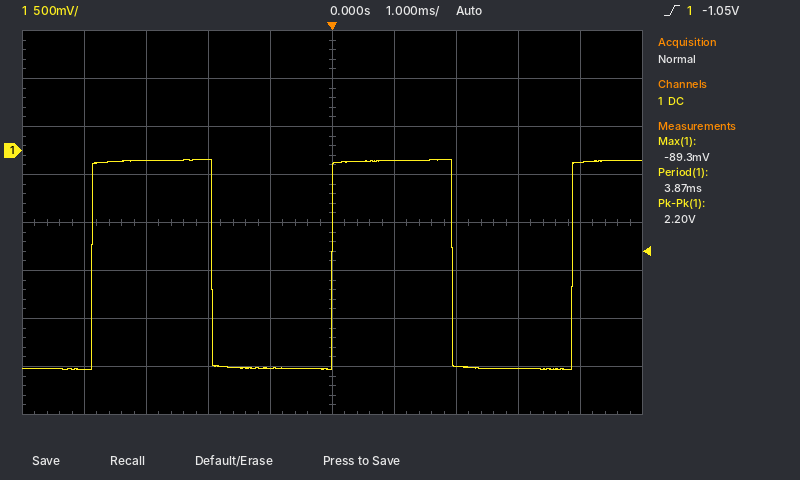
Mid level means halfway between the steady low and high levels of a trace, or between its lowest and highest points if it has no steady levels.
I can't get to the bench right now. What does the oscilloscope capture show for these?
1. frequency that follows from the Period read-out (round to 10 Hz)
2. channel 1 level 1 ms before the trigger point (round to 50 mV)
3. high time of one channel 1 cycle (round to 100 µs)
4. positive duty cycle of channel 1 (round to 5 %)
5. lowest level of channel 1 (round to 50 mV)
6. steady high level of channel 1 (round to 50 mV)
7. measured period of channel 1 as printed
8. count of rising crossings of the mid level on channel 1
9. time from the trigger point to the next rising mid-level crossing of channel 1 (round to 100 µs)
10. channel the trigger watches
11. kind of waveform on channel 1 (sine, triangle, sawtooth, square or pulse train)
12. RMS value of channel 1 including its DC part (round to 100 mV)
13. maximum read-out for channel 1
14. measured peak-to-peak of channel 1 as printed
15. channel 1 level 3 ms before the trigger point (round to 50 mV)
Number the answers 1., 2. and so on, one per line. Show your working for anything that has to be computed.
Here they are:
1. 1 / 3.87 ms ≈ 258 Hz, so 260 Hz to the nearest 10 Hz
2. -2.25 V
3. 1.9 ms
4. 50 %
5. -2.30 V
6. -100 mV
7. 3.87 ms
8. 3
9. 3.9 ms
10. channel 1
11. square
12. √(0.5 × (-100 mV)² + 0.5 × (-2.30 V)²) ≈ 1.6 V
13. -89.3 mV
14. 2.20 V
15. -100 mV
